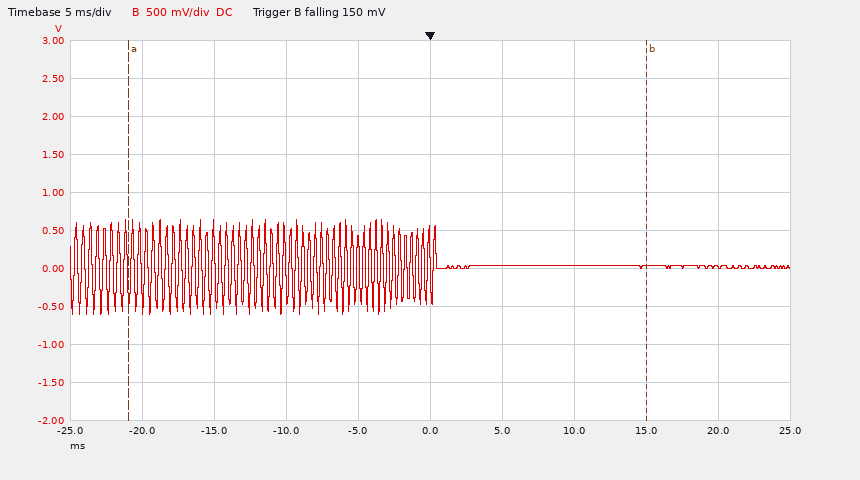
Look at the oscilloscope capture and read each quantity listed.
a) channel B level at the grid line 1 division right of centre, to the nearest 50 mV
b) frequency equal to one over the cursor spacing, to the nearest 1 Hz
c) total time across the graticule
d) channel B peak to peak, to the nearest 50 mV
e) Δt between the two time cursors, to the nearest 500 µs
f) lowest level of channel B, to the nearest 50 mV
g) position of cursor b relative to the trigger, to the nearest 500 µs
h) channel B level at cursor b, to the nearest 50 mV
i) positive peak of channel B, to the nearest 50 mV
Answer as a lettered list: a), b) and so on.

a) 50 mV
b) 28 Hz
c) 50 ms
d) 1.25 V
e) 36.0 ms
f) -600 mV
g) +15.0 ms
h) 50 mV
i) 650 mV
